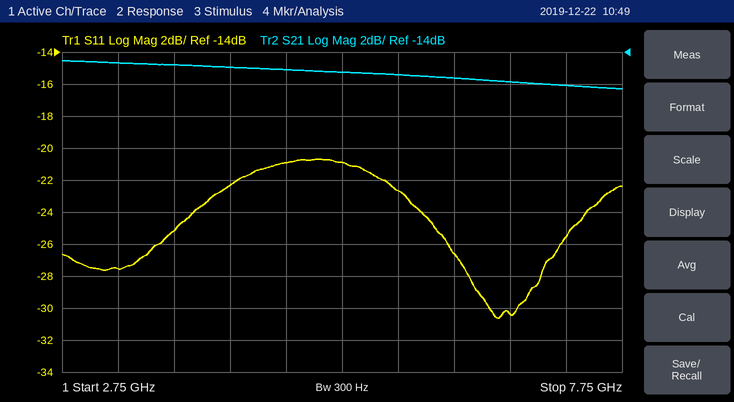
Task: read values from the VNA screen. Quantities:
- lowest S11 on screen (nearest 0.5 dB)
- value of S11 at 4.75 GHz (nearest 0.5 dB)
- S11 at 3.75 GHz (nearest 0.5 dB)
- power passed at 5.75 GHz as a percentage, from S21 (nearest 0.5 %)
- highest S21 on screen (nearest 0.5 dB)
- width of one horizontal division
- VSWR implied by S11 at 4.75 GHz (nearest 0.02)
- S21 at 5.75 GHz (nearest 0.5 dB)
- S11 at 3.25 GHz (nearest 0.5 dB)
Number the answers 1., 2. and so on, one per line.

1. -30.5 dB
2. -21.0 dB
3. -25.0 dB
4. 3.0 %
5. -14.5 dB
6. 500 MHz
7. 1.20
8. -15.5 dB
9. -27.5 dB
